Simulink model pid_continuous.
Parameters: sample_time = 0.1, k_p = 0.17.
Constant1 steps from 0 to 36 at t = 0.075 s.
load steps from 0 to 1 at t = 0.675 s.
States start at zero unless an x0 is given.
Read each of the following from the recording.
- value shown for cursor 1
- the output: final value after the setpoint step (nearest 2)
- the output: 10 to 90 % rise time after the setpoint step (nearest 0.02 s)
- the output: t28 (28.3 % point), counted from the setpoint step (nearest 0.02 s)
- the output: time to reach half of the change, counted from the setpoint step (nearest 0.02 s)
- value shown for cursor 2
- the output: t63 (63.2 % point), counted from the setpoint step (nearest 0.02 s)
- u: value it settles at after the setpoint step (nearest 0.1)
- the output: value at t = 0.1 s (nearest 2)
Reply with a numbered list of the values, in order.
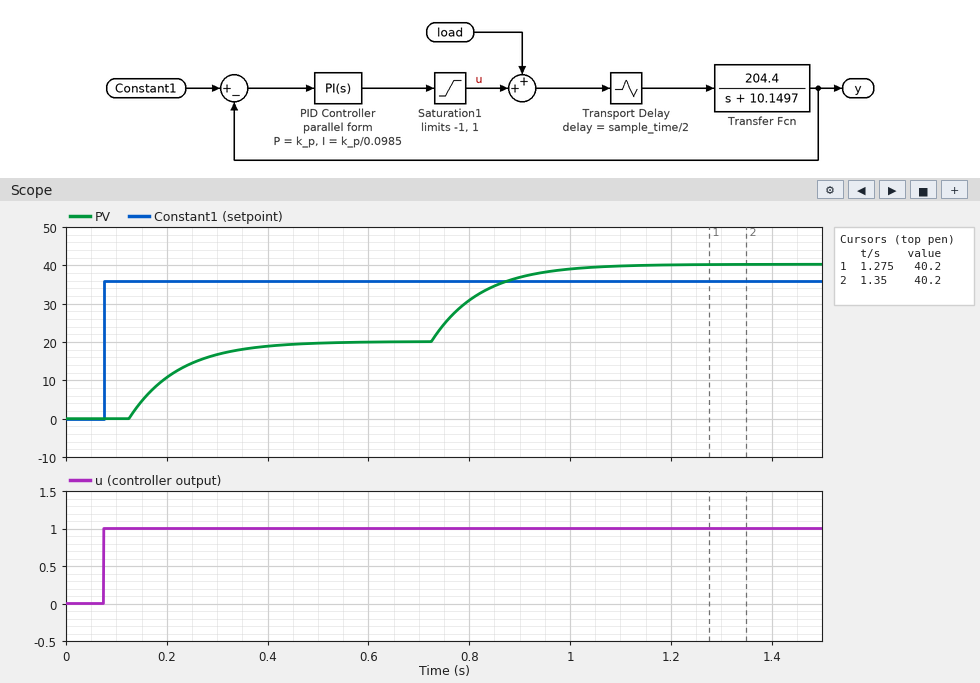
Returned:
1. 40.2
2. 20
3. 0.22 s
4. 0.08 s
5. 0.12 s
6. 40.2
7. 0.14 s
8. 1.0
9. 0
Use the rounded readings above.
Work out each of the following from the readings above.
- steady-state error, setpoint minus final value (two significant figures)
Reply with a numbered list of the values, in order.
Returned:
1. 16
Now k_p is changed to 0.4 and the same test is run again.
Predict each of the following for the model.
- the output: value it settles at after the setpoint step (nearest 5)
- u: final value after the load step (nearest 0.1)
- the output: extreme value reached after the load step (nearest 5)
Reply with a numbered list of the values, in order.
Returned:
1. 20
2. 1.0
3. 40
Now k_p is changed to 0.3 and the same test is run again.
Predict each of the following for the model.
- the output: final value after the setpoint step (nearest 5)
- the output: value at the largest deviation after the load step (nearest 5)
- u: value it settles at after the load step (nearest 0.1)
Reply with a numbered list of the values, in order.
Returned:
1. 20
2. 40
3. 1.0
